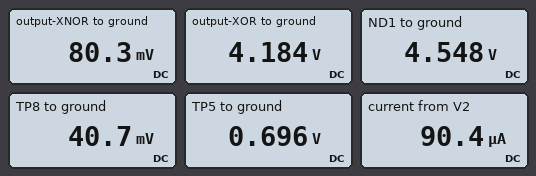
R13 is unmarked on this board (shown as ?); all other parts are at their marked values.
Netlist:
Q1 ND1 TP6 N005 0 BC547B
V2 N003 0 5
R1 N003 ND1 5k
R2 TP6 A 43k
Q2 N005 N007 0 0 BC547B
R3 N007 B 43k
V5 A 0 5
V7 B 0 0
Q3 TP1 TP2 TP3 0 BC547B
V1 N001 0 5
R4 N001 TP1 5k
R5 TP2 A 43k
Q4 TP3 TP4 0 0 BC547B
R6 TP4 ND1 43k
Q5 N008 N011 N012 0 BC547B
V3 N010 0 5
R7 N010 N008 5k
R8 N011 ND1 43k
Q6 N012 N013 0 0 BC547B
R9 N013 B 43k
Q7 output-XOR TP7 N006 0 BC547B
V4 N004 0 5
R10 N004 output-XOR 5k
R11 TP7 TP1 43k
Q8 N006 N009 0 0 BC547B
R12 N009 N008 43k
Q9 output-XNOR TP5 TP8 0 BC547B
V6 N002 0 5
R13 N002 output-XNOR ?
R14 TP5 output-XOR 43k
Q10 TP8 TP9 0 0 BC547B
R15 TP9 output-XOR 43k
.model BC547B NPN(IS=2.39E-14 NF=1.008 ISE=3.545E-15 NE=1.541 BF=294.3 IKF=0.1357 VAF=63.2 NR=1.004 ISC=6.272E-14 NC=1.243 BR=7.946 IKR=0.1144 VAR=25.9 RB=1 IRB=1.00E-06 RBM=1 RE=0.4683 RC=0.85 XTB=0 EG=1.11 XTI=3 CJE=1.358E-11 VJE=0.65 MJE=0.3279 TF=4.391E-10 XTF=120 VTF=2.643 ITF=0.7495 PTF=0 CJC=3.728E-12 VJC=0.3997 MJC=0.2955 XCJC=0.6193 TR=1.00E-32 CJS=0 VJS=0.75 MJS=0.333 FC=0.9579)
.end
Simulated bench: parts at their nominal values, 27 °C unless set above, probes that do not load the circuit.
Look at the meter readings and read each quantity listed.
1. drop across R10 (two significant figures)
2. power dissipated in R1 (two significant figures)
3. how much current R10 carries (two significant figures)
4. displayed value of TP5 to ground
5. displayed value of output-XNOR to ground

820 mV
41 µW
160 µA
0.696 V
80.3 mV
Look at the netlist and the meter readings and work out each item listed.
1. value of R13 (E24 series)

3.9 kΩ
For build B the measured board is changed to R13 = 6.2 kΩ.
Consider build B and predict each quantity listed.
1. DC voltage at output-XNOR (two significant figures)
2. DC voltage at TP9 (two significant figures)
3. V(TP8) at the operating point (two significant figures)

63 mV
650 mV
32 mV
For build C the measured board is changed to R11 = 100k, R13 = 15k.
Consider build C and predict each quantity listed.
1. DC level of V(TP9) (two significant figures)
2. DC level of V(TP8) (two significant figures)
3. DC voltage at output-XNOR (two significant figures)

640 mV
21 mV
40 mV
